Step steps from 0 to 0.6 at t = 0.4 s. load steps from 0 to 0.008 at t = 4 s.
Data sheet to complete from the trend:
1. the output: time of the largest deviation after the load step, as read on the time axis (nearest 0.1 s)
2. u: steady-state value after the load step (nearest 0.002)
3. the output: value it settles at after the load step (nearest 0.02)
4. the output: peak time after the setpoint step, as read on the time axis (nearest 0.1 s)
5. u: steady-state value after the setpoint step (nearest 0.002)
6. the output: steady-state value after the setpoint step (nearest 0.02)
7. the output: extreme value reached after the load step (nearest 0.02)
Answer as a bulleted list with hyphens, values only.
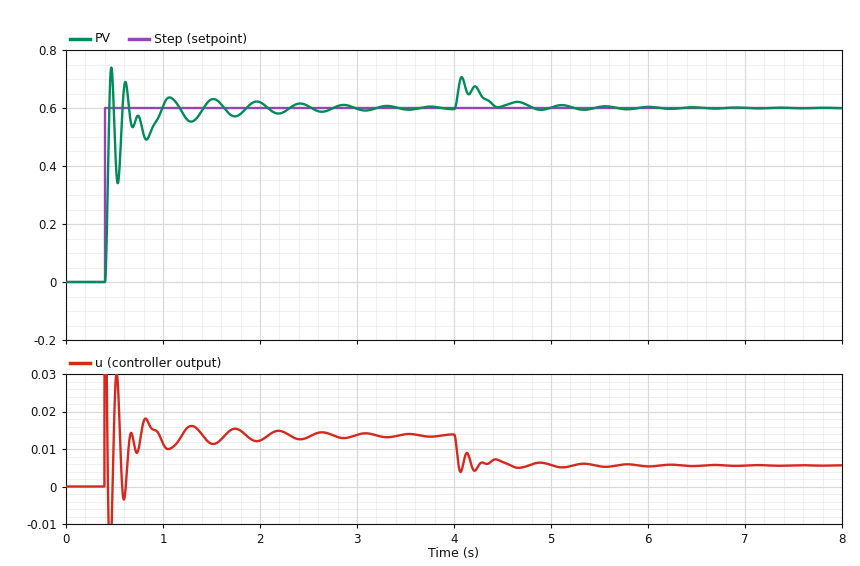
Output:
- 4.1 s
- 0.006
- 0.60
- 0.5 s
- 0.014
- 0.60
- 0.70
